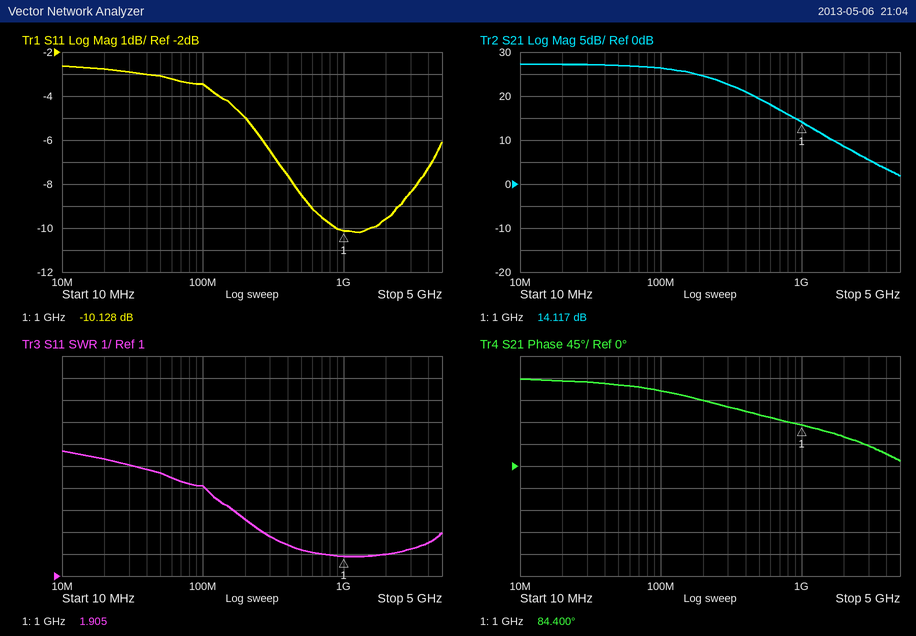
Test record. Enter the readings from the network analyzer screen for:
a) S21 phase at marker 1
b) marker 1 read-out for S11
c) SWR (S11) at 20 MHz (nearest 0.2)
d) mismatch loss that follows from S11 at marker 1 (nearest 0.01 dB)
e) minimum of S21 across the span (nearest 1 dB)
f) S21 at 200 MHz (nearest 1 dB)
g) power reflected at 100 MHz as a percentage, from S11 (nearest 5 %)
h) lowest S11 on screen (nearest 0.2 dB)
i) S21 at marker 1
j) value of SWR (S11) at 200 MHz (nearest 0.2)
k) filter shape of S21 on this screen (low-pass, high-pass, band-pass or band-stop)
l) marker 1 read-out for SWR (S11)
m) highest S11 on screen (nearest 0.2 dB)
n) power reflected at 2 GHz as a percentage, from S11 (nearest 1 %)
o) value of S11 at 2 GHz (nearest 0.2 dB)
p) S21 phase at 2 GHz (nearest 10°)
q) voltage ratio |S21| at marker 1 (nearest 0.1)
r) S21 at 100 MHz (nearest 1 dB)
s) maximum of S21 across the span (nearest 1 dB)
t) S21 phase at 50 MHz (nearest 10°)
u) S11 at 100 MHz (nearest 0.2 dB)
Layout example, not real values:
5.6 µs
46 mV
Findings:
84.400°
-10.128 dB
6.4
0.44 dB
2 dB
25 dB
45 %
-10.2 dB
14.117 dB
3.6
low-pass
1.905
-2.6 dB
11 %
-9.6 dB
60°
5.1
26 dB
27 dB
170°
-3.4 dB
